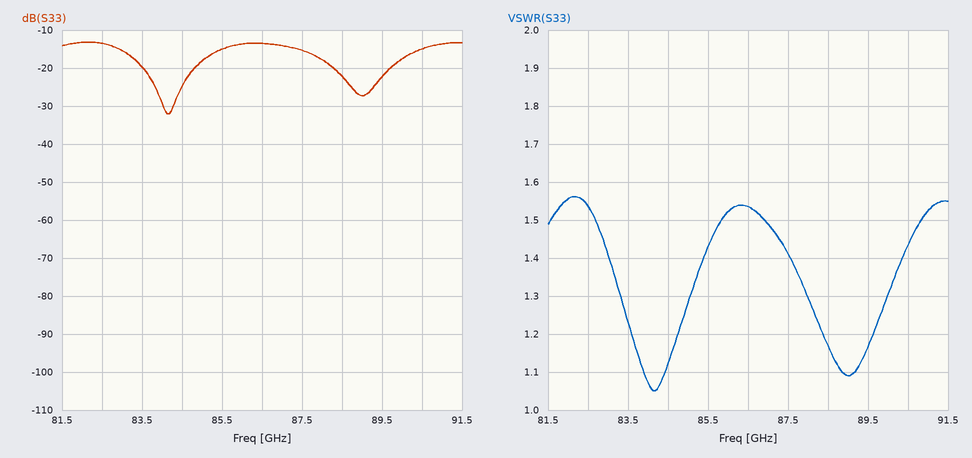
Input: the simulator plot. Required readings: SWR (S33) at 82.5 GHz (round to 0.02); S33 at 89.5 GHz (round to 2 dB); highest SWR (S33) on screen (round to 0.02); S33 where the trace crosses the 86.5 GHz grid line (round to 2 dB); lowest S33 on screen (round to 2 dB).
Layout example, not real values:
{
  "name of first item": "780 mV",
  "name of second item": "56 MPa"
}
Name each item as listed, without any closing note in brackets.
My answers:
{
  "SWR (S33) at 82.5 GHz": "1.54",
  "S33 at 89.5 GHz": "-22 dB",
  "highest SWR (S33) on screen": "1.56",
  "S33 where the trace crosses the 86.5 GHz grid line": "-14 dB",
  "lowest S33 on screen": "-32 dB"
}
